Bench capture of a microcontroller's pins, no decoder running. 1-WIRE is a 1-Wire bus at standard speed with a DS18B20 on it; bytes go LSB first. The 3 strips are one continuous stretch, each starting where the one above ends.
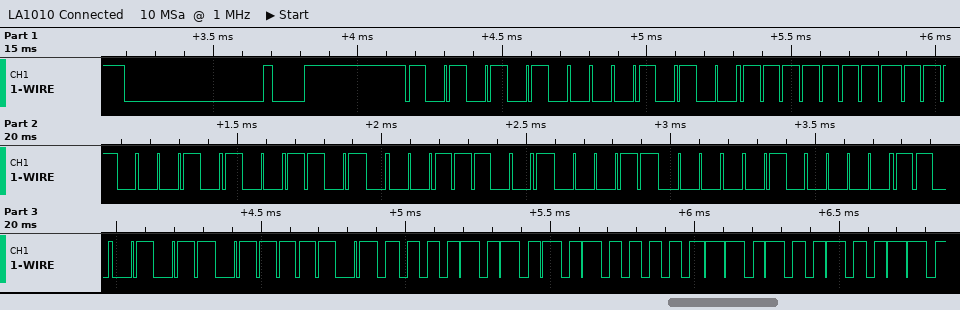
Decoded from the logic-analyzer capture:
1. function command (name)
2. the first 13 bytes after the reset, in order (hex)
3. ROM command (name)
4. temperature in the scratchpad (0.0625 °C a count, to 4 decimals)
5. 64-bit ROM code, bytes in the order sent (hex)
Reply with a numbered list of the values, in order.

1. Read Scratchpad
2. 55 28 FF 47 59 9C 18 04 D3 BE 50 05 4B
3. Match ROM
4. 85.0000 °C
5. 28 FF 47 59 9C 18 04 D3
